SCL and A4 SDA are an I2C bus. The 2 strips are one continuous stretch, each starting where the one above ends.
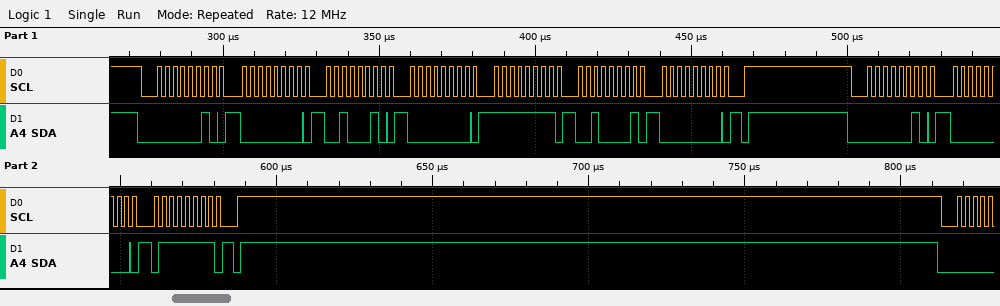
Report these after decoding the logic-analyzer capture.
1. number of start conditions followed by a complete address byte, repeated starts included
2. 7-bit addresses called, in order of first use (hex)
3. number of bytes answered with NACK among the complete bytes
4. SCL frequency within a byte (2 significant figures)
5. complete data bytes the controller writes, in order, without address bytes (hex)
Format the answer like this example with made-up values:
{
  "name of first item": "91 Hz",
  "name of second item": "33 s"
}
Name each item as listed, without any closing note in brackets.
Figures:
{
  "number of start conditions followed by a complete address byte, repeated starts included": "2",
  "7-bit addresses called, in order of first use": "0x01",
  "number of bytes answered with NACK among the complete bytes": "0",
  "SCL frequency within a byte": "400 kHz",
  "complete data bytes the controller writes, in order, without address bytes": "00 22 00 FF 21 00 00 7F"
}
